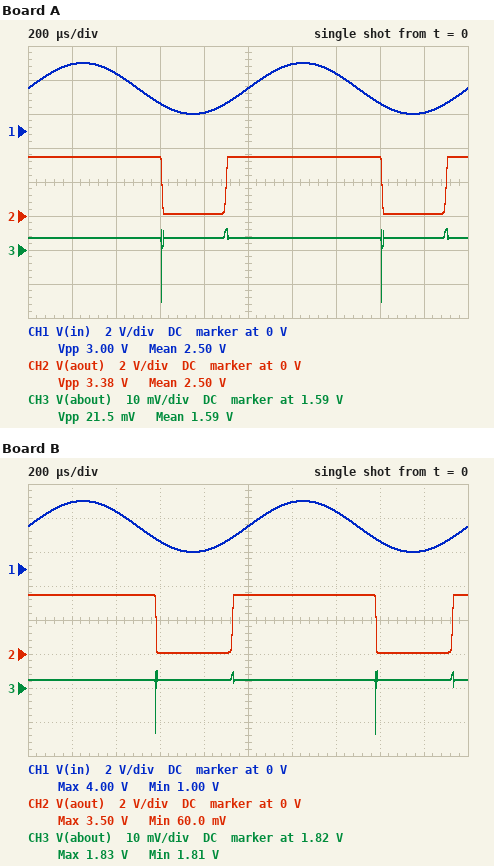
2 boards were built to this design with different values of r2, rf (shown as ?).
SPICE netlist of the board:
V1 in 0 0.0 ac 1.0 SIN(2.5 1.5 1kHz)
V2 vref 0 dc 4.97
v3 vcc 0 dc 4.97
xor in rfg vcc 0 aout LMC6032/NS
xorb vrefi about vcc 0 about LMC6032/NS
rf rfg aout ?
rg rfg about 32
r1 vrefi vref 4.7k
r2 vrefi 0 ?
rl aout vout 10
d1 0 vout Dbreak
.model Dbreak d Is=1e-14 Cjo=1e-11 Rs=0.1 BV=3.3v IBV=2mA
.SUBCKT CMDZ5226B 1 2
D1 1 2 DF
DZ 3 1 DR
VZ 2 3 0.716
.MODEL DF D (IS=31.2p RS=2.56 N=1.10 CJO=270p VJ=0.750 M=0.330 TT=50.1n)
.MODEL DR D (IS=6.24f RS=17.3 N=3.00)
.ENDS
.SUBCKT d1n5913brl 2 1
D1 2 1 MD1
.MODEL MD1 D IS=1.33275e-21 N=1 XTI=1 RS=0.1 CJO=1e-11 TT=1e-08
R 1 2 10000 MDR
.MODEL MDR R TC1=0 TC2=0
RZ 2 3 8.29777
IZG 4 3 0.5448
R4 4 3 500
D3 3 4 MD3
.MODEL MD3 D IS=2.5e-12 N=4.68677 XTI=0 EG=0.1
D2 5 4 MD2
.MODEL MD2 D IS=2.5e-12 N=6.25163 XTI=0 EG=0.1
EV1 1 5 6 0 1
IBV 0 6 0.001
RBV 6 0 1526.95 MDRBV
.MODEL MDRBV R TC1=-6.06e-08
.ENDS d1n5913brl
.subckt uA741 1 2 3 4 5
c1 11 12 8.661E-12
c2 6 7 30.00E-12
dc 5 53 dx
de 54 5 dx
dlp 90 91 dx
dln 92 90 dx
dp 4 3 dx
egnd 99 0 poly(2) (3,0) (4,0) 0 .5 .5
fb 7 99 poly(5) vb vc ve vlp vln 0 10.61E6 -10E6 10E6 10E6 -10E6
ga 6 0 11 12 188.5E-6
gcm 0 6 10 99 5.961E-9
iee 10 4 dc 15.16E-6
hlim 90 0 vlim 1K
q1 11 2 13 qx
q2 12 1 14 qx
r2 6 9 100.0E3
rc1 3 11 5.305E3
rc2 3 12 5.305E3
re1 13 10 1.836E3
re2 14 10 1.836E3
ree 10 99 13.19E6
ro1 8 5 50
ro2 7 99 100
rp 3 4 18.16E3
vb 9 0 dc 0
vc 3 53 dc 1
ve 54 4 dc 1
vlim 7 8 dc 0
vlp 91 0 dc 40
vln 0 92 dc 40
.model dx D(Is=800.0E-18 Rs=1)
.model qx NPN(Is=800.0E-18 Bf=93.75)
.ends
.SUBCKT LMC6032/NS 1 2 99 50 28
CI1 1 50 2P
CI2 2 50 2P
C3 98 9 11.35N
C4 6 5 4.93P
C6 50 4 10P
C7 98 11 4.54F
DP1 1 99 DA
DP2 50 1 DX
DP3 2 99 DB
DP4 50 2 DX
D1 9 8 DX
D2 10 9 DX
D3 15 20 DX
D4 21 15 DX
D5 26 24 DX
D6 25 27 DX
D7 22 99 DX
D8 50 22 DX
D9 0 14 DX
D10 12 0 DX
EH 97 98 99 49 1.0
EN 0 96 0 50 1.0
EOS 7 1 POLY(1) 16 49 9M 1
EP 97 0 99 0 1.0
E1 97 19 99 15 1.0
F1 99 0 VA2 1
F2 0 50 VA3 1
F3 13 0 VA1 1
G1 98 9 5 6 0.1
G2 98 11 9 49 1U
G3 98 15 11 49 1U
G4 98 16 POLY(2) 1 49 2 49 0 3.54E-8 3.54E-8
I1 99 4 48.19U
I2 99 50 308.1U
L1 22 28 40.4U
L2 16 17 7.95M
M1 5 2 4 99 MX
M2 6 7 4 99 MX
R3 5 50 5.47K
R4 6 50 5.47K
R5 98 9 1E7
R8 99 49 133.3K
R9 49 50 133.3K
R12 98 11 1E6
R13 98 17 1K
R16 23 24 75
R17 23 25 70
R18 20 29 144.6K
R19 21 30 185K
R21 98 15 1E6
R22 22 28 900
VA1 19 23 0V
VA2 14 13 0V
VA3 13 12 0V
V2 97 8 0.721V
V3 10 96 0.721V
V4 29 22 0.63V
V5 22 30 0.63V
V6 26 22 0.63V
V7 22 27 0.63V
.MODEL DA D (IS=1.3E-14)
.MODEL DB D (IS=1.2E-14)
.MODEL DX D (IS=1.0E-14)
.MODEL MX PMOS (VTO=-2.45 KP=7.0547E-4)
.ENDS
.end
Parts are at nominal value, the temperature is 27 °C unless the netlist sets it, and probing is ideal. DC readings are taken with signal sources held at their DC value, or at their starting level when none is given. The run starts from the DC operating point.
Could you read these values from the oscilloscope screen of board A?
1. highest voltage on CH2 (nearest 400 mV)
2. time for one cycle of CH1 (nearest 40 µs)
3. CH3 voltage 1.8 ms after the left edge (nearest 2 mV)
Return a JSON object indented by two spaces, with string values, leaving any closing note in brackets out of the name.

{
  "highest voltage on CH2": "3.6 V",
  "time for one cycle of CH1": "1.00 ms",
  "CH3 voltage 1.8 ms after the left edge": "1.594 V"
}
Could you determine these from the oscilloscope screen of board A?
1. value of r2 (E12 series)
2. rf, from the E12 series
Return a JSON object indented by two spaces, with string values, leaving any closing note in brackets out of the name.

{
  "value of r2": "2.2 kΩ",
  "rf, from the E12 series": "1.2 kΩ"
}
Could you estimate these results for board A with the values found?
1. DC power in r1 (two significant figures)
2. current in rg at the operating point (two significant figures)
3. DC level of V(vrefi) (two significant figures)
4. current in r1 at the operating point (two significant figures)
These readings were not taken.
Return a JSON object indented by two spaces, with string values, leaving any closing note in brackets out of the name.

{
  "DC power in r1": "2.4 mW",
  "current in rg at the operating point": "1.2 mA",
  "DC level of V(vrefi)": "1.6 V",
  "current in r1 at the operating point": "720 µA"
}
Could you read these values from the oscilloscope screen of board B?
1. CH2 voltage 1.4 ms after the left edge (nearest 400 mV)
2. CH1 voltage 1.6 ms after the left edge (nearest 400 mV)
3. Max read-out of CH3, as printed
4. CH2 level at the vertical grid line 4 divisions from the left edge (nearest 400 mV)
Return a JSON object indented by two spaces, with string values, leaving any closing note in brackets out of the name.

{
  "CH2 voltage 1.4 ms after the left edge": "3.6 V",
  "CH1 voltage 1.6 ms after the left edge": "1.6 V",
  "Max read-out of CH3, as printed": "1.83 V",
  "CH2 level at the vertical grid line 4 divisions from the left edge": "0 V"
}
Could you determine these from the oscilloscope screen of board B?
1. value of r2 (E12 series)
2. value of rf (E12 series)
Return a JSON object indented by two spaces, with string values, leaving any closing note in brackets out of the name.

{
  "value of r2": "2.7 kΩ",
  "value of rf": "2.2 kΩ"
}
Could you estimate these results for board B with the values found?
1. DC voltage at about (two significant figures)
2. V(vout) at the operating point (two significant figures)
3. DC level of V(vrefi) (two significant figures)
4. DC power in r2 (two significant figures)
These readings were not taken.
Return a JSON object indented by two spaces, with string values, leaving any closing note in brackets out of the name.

{
  "DC voltage at about": "1.8 V",
  "V(vout) at the operating point": "61 mV",
  "DC level of V(vrefi)": "1.8 V",
  "DC power in r2": "1.2 mW"
}
